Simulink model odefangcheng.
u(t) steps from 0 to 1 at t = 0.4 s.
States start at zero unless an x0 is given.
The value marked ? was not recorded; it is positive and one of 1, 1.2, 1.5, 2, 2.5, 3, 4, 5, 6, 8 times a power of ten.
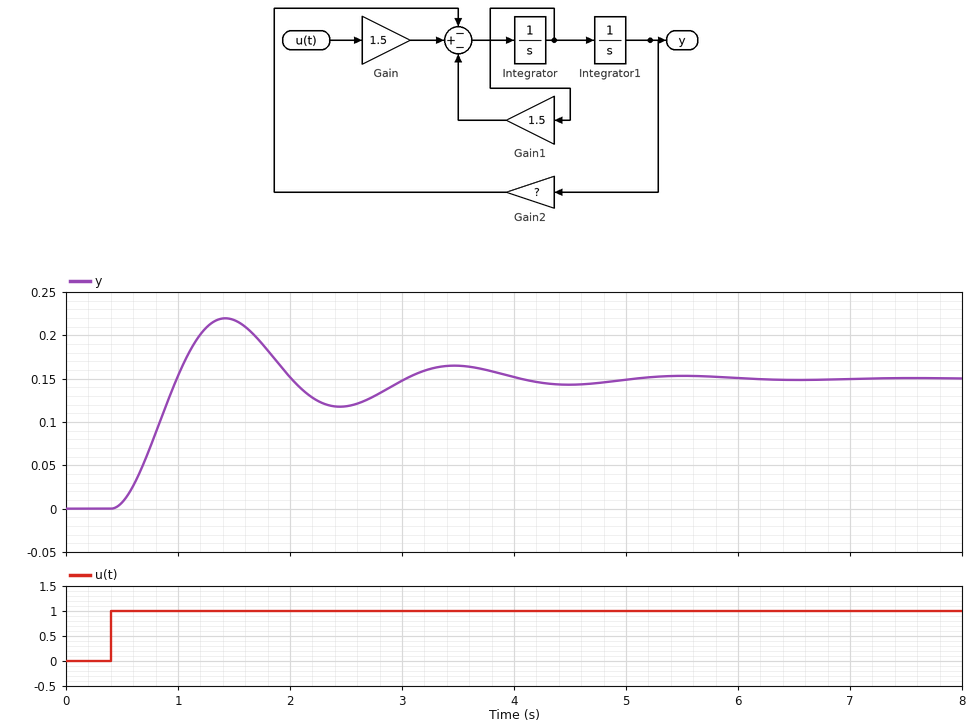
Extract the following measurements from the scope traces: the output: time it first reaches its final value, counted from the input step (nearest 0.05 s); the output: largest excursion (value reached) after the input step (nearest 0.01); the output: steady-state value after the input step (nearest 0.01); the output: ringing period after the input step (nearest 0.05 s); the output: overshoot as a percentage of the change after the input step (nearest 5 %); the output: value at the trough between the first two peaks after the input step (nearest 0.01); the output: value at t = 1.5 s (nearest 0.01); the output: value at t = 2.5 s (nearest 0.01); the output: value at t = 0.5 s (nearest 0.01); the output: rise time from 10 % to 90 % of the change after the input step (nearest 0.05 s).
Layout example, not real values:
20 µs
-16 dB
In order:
0.60 s
0.22
0.15
2.05 s
45 %
0.12
0.22
0.12
0.01
0.40 s
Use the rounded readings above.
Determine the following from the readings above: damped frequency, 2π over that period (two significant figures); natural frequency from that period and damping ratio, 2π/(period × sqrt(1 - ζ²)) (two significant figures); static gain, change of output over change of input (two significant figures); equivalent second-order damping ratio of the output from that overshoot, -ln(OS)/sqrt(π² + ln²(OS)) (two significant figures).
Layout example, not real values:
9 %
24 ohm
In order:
3.1 rad/s
3.2 rad/s
0.15
0.25
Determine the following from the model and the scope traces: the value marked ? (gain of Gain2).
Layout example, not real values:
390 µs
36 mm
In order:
10
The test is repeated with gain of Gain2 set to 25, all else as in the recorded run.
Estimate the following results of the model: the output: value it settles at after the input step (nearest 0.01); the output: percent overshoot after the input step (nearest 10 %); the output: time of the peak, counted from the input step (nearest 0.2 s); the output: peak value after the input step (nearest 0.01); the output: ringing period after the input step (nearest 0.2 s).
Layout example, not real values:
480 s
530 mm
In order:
0.06
60 %
0.6 s
0.10
1.2 s
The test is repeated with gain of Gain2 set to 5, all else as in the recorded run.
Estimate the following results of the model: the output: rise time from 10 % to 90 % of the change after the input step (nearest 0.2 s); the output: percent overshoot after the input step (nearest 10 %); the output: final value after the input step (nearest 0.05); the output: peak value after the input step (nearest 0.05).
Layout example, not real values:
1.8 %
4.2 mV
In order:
0.6 s
30 %
0.30
0.40
